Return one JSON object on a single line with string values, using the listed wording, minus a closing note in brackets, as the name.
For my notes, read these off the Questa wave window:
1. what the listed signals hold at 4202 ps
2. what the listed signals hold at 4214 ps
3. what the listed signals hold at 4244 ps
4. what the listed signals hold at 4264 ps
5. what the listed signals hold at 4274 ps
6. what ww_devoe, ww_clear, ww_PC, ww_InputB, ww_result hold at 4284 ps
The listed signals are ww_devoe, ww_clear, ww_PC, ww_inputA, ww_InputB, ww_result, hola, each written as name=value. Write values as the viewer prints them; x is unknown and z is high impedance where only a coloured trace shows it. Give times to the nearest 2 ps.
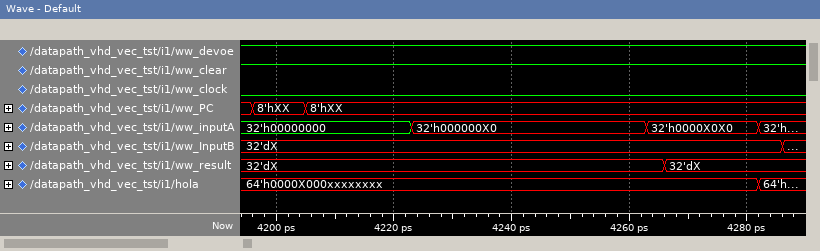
{"what the listed signals hold at 4202 ps": "ww_devoe=1, ww_clear=1, ww_PC=8'hXX, ww_inputA=32'h00000000, ww_InputB=32'dX, ww_result=32'dX, hola=64'h0000X000xxxxxxxx", "what the listed signals hold at 4214 ps": "ww_devoe=1, ww_clear=1, ww_PC=8'hXX, ww_inputA=32'h00000000, ww_InputB=32'dX, ww_result=32'dX, hola=64'h0000X000xxxxxxxx", "what the listed signals hold at 4244 ps": "ww_devoe=1, ww_clear=1, ww_PC=8'hXX, ww_inputA=32'h000000X0, ww_InputB=32'dX, ww_result=32'dX, hola=64'h0000X000xxxxxxxx", "what the listed signals hold at 4264 ps": "ww_devoe=1, ww_clear=1, ww_PC=8'hXX, ww_inputA=32'h0000X0X0, ww_InputB=32'dX, ww_result=32'dX, hola=64'h0000X000xxxxxxxx", "what the listed signals hold at 4274 ps": "ww_devoe=1, ww_clear=1, ww_PC=8'hXX, ww_inputA=32'h0000X0X0, ww_InputB=32'dX, ww_result=32'dX, hola=64'h0000X000xxxxxxxx", "what ww_devoe, ww_clear, ww_PC, ww_InputB, ww_result hold at 4284 ps": "ww_devoe=1, ww_clear=1, ww_PC=8'hXX, ww_InputB=32'dX, ww_result=32'dX"}
